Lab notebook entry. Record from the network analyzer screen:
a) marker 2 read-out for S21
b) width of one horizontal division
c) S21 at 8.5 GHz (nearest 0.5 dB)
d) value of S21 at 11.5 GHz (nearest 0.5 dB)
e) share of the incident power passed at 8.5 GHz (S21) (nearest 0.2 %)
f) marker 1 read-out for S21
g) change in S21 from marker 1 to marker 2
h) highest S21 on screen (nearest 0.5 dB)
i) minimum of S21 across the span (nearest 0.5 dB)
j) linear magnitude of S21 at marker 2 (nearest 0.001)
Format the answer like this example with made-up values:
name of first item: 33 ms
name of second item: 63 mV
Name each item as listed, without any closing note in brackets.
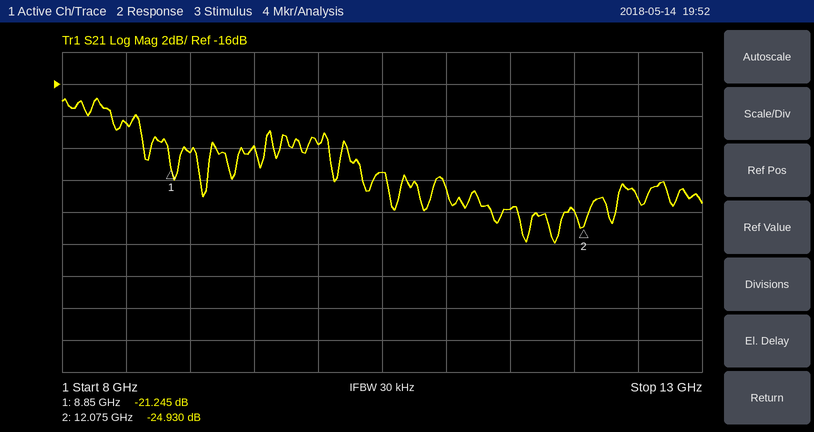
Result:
marker 2 read-out for S21: -24.930 dB
width of one horizontal division: 500 MHz
S21 at 8.5 GHz: -18.5 dB
value of S21 at 11.5 GHz: -24.0 dB
share of the incident power passed at 8.5 GHz (S21): 1.4 %
marker 1 read-out for S21: -21.245 dB
change in S21 from marker 1 to marker 2: -3.685 dB
highest S21 on screen: -17.0 dB
minimum of S21 across the span: -26.0 dB
linear magnitude of S21 at marker 2: 0.057
